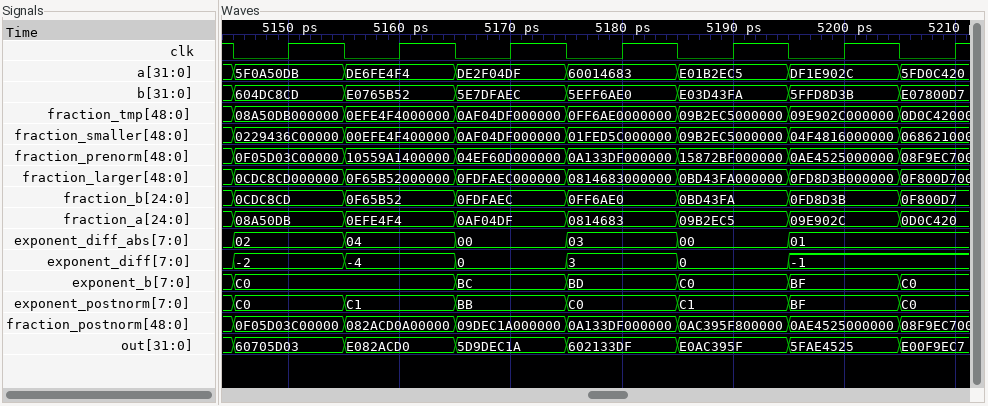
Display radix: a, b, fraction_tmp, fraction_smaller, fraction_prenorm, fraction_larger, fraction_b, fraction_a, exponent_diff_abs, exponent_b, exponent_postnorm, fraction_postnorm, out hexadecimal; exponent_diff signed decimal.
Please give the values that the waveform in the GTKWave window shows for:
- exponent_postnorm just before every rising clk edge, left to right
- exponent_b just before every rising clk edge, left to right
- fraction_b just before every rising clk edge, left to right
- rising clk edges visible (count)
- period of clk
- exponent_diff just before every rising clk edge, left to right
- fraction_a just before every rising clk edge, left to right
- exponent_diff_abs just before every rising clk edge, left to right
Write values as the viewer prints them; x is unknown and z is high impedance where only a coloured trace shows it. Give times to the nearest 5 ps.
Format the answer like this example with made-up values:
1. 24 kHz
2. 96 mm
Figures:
1. C0, C1, BB, C0, C1, BF, C0
2. C0, C0, BC, BD, C0, BF, C0
3. 0CDC8CD, 0F65B52, 0FDFAEC, 0FF6AE0, 0BD43FA, 0FD8D3B, 0F800D7
4. 7
5. 10 ps
6. -2, -4, 0, 3, 0, -1, -1
7. 08A50DB, 0EFE4F4, 0AF04DF, 0814683, 09B2EC5, 09E902C, 0D0C420
8. 02, 04, 00, 03, 00, 01, 01
